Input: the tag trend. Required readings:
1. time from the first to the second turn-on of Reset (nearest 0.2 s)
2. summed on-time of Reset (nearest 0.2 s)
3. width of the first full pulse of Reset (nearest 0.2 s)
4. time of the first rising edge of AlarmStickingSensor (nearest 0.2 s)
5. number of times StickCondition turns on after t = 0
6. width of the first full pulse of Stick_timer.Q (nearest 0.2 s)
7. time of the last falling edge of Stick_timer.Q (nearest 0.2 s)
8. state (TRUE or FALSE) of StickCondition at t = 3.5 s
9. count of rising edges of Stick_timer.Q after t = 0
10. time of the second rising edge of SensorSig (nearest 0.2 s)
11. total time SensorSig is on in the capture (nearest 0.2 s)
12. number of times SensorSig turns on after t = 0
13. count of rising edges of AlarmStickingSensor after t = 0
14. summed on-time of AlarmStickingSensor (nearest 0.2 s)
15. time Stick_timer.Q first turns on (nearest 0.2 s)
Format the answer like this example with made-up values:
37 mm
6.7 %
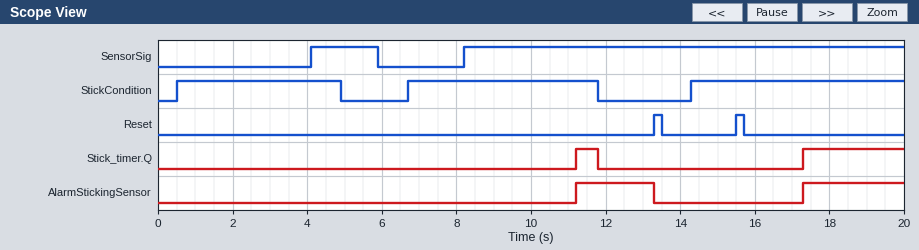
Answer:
2.2 s
0.4 s
0.2 s
11.2 s
3
0.6 s
11.8 s
TRUE
2
8.2 s
13.6 s
2
2
4.8 s
11.2 s
